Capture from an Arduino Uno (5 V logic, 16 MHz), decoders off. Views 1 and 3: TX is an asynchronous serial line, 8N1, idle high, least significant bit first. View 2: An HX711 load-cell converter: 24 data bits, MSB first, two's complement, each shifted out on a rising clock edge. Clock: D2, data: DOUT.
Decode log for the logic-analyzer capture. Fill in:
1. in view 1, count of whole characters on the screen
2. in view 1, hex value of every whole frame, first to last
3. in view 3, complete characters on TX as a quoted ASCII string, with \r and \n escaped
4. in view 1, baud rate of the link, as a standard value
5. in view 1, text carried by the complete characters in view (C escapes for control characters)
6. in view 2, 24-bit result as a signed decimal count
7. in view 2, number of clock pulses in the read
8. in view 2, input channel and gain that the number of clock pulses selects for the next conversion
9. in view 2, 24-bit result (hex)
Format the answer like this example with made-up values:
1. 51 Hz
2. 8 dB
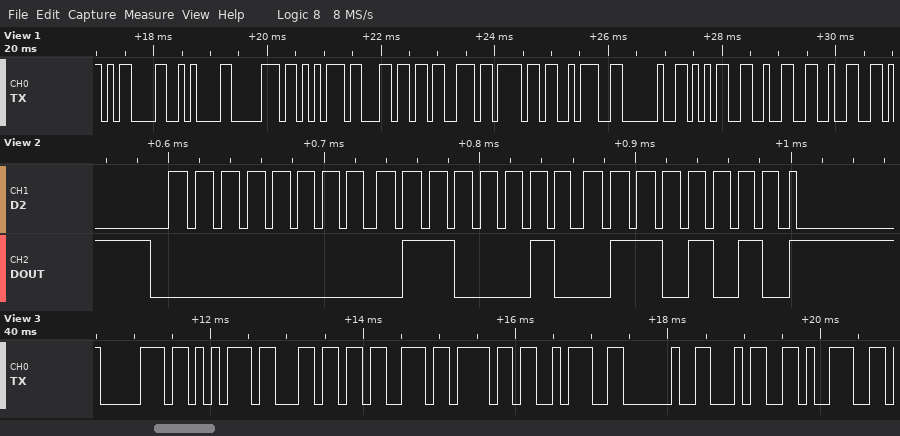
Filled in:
1. 12
2. 0x0D 0x0A 0x70 0x75 0x6C 0x73 0x6F 0x3A 0x20 0x35 0x32 0x32
3. "pulso: 49"
4. 9600 baud
5. "\r\npulso: 522"
6. 25194
7. 25
8. channel A, gain 128
9. 0x00626A
